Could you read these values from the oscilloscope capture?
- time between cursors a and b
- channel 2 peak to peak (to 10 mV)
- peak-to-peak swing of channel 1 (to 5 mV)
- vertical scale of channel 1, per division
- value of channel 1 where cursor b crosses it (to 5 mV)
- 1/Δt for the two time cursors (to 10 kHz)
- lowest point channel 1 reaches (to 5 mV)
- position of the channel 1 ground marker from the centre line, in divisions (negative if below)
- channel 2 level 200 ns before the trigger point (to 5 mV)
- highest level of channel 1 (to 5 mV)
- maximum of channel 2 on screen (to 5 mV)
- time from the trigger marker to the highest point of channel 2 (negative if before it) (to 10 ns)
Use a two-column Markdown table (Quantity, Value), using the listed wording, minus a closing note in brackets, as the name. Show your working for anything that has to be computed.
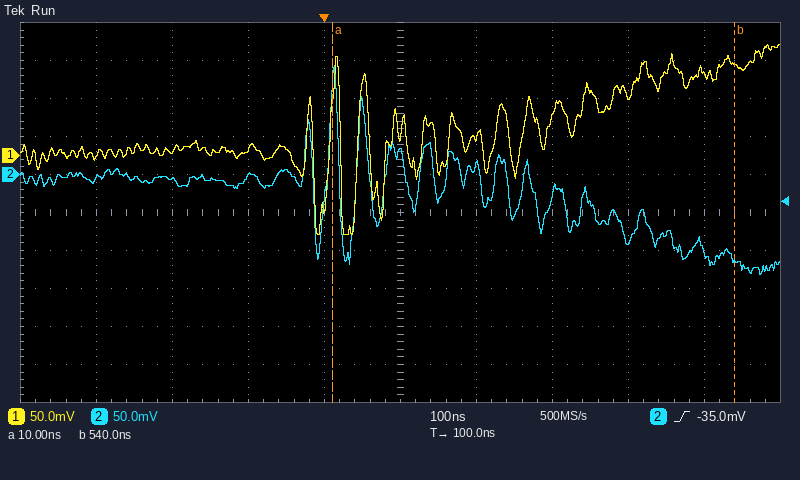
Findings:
| Quantity | Value |
|---|---|
| time between cursors a and b | 540 ns − (10 ns) = 530 ns |
| channel 2 peak to peak | 280 mV |
| peak-to-peak swing of channel 1 | 145 mV − (-105 mV) = 250 mV |
| vertical scale of channel 1, per division | 50 mV |
| value of channel 1 where cursor b crosses it | 120 mV |
| 1/Δt for the two time cursors | 1 / 530 ns ≈ 1.89 MHz |
| lowest point channel 1 reaches | -105 mV |
| position of the channel 1 ground marker from the centre line, in divisions | +1.5 div |
| channel 2 level 200 ns before the trigger point | -5 mV |
| highest level of channel 1 | 145 mV |
| maximum of channel 2 on screen | 145 mV |
| time from the trigger marker to the highest point of channel 2 (negative if before it) | +10 ns |
